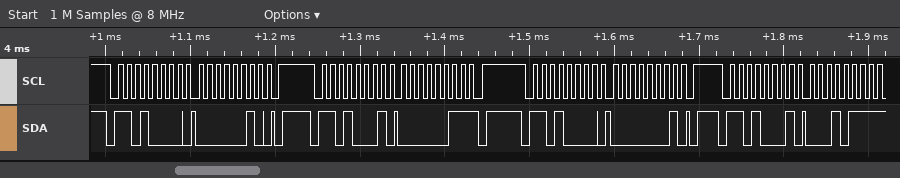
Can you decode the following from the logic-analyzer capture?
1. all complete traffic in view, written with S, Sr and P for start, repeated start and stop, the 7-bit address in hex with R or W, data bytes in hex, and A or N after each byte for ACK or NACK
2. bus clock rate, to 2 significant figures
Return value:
S 68W A 02 A P S 68R A 03 N P S 68W A 01 A P S 68R A 17 N
100 kHz
